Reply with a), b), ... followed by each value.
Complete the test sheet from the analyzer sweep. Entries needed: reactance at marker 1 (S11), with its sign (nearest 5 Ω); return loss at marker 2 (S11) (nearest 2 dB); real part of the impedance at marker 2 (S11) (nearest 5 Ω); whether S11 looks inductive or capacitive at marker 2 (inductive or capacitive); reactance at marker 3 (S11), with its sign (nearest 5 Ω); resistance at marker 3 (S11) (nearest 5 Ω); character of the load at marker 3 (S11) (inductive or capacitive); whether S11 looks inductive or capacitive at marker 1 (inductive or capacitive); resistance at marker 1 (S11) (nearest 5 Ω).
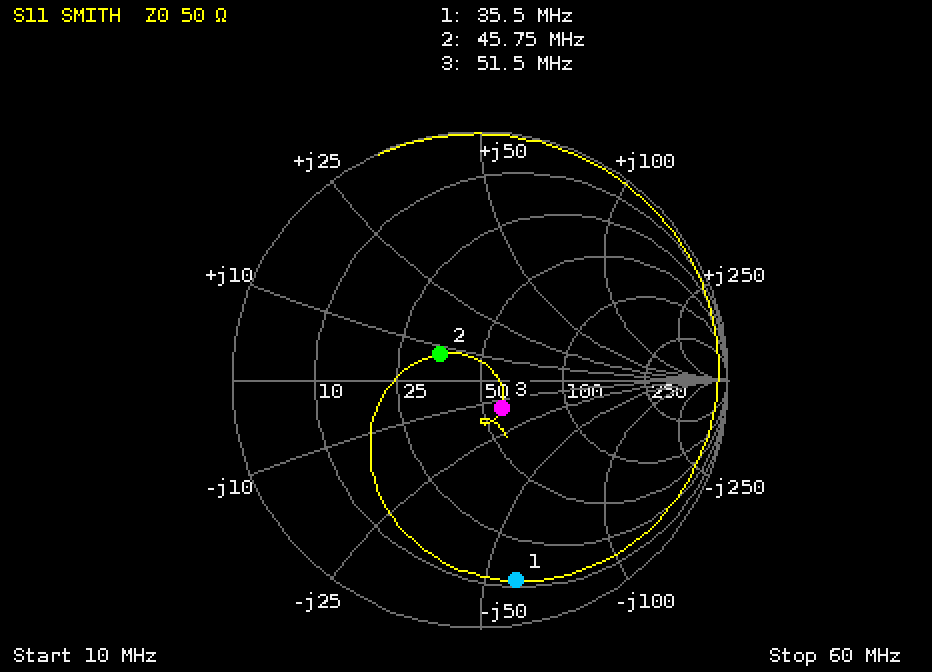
a) -60 Ω
b) 14 dB
c) 35 Ω
d) inductive
e) -15 Ω
f) 60 Ω
g) capacitive
h) capacitive
i) 10 Ω
